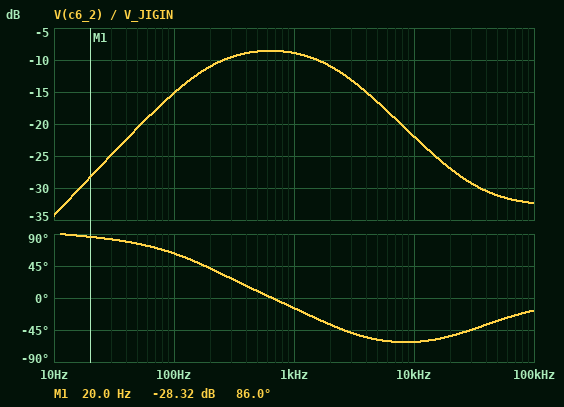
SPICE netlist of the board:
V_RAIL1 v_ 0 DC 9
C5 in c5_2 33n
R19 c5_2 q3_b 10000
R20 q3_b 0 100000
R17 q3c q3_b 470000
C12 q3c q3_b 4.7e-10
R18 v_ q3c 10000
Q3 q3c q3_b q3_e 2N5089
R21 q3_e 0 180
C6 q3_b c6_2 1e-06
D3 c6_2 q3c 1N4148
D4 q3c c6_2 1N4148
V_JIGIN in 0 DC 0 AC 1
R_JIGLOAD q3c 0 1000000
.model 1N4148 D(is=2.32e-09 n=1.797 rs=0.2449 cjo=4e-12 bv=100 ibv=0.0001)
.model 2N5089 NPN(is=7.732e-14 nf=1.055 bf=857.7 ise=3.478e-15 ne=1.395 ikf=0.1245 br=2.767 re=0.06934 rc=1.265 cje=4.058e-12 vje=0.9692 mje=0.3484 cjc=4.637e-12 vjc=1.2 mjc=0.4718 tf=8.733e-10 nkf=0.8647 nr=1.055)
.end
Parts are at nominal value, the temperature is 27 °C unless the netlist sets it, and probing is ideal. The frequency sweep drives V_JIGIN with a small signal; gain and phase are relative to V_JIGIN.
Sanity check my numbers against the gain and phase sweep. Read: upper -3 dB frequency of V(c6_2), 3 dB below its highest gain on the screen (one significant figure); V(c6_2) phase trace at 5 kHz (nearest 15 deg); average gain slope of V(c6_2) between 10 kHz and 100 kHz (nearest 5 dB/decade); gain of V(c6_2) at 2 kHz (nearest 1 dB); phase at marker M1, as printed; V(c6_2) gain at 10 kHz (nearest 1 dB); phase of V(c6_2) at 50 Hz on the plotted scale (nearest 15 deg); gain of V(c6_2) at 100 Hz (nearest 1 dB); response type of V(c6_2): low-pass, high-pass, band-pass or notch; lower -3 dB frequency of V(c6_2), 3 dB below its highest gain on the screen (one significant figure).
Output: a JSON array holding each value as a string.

["2 kHz", "-60 deg", "-10 dB/decade", "-11 dB", "86.0 deg", "-22 dB", "75 deg", "-15 dB", "band-pass", "200 Hz"]
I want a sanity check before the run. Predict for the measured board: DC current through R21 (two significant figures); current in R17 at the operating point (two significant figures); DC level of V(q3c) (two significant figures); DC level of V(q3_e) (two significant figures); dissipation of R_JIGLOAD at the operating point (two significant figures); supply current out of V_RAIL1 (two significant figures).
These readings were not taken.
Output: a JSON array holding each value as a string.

["460 µA", "7.6 µA", "4.3 V", "83 mV", "18 µW", "470 µA"]
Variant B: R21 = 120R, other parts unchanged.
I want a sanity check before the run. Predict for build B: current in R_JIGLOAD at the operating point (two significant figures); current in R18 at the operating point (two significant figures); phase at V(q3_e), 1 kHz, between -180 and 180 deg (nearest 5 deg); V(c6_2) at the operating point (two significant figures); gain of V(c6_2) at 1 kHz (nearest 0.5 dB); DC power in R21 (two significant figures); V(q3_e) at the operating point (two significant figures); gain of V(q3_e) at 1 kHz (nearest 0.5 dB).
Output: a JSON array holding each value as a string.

["4.1 µA", "490 µA", "-15 deg", "4.1 V", "-10.5 dB", "27 µW", "57 mV", "-14.0 dB"]
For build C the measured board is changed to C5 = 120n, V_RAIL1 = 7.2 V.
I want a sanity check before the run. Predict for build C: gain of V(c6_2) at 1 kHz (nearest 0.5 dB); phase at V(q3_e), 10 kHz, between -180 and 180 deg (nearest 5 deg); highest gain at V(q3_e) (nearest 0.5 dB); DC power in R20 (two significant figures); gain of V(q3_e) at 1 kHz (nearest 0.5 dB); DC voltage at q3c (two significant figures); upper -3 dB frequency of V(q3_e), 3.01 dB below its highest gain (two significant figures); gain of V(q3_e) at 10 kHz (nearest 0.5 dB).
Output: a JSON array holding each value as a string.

["-7.5 dB", "-65 deg", "-10.0 dB", "4.4 µW", "-11.0 dB", "4.0 V", "1.9 kHz", "-24.5 dB"]
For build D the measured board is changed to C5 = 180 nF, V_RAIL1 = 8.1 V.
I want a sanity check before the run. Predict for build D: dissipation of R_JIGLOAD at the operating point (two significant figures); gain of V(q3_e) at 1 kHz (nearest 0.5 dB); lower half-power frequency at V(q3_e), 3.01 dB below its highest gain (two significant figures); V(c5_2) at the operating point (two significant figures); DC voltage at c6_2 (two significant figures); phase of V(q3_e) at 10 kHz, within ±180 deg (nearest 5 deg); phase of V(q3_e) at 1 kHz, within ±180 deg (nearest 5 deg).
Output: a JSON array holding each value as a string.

["17 µW", "-10.5 dB", "42 Hz", "680 mV", "4.1 V", "-65 deg", "-25 deg"]
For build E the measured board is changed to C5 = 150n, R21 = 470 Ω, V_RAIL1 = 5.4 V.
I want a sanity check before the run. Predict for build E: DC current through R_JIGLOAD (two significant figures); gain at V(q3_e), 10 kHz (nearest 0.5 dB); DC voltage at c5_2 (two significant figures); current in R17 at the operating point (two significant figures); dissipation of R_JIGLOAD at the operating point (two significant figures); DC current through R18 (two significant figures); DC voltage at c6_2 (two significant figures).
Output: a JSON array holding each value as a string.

["3.8 µA", "-17.0 dB", "650 mV", "6.7 µA", "15 µW", "160 µA", "3.8 V"]
